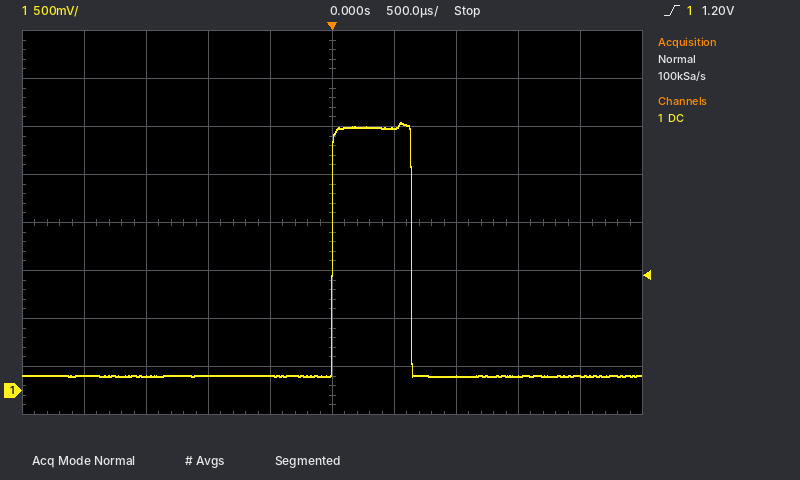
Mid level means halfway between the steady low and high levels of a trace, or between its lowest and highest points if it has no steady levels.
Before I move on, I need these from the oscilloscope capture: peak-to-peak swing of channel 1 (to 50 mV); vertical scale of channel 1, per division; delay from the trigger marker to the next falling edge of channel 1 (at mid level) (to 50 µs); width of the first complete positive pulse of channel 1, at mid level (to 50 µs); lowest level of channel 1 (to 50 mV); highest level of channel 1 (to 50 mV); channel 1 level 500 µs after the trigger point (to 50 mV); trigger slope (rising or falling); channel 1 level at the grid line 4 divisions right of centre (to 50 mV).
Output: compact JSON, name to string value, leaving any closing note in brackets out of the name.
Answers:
{"peak-to-peak swing of channel 1": "2.65 V", "vertical scale of channel 1, per division": "500 mV", "delay from the trigger marker to the next falling edge of channel 1 (at mid level)": "650 µs", "width of the first complete positive pulse of channel 1, at mid level": "650 µs", "lowest level of channel 1": "150 mV", "highest level of channel 1": "2.80 V", "channel 1 level 500 µs after the trigger point": "2.75 V", "trigger slope": "rising", "channel 1 level at the grid line 4 divisions right of centre": "150 mV"}
